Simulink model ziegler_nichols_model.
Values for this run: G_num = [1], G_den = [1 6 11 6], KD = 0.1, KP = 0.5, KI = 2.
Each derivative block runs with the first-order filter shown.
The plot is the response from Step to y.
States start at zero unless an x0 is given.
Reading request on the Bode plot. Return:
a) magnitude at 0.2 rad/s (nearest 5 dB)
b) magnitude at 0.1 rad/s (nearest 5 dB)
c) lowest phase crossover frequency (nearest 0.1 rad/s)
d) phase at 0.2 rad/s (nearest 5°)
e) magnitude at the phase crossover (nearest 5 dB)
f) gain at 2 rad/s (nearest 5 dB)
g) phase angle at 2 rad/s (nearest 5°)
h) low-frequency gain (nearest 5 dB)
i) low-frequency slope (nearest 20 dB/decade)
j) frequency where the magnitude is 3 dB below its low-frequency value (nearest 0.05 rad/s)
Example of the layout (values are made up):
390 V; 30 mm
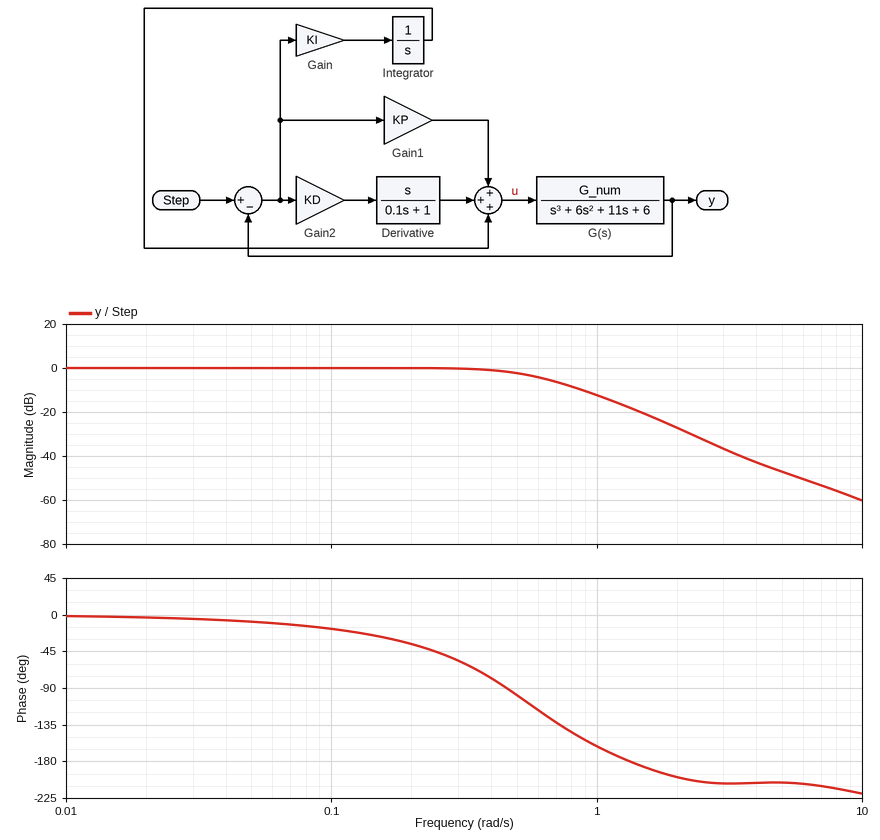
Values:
0 dB; 0 dB; 1.3 rad/s; -35°; -20 dB; -25 dB; -200°; 0 dB; 0 dB/decade; 0.55 rad/s
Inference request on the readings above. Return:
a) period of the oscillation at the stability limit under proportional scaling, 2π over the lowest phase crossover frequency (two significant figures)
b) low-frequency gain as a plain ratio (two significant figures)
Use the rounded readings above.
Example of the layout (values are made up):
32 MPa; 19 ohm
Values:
4.8 s; 1.0
